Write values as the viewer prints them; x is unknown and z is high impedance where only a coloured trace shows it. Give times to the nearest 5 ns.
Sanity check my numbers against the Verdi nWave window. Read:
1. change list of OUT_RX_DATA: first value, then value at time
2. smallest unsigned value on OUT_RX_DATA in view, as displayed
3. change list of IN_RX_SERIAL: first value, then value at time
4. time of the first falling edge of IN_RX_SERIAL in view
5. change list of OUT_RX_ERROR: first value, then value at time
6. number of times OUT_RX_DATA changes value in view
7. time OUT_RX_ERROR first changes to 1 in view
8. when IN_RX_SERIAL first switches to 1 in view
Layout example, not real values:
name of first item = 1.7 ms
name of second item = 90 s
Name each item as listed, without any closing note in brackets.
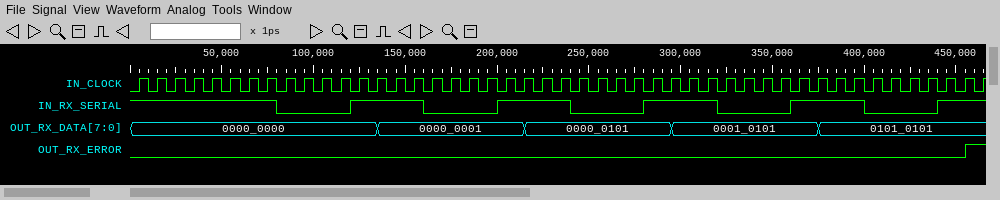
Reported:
change list of OUT_RX_DATA: first value, then value at time = 0000_0000, 0000_0001 at 135 ns, 0000_0101 at 215 ns, 0001_0101 at 295 ns, 0101_0101 at 375 ns
smallest unsigned value on OUT_RX_DATA in view, as displayed = 0000_0000
change list of IN_RX_SERIAL: first value, then value at time = 1, 0 at 80 ns, 1 at 120 ns, 0 at 160 ns, 1 at 200 ns, 0 at 240 ns, 1 at 280 ns, 0 at 320 ns, 1 at 360 ns, 0 at 400 ns, 1 at 440 ns
time of the first falling edge of IN_RX_SERIAL in view = 80 ns
change list of OUT_RX_ERROR: first value, then value at time = 0, 1 at 455 ns
number of times OUT_RX_DATA changes value in view = 4
time OUT_RX_ERROR first changes to 1 in view = 455 ns
when IN_RX_SERIAL first switches to 1 in view = 120 ns
